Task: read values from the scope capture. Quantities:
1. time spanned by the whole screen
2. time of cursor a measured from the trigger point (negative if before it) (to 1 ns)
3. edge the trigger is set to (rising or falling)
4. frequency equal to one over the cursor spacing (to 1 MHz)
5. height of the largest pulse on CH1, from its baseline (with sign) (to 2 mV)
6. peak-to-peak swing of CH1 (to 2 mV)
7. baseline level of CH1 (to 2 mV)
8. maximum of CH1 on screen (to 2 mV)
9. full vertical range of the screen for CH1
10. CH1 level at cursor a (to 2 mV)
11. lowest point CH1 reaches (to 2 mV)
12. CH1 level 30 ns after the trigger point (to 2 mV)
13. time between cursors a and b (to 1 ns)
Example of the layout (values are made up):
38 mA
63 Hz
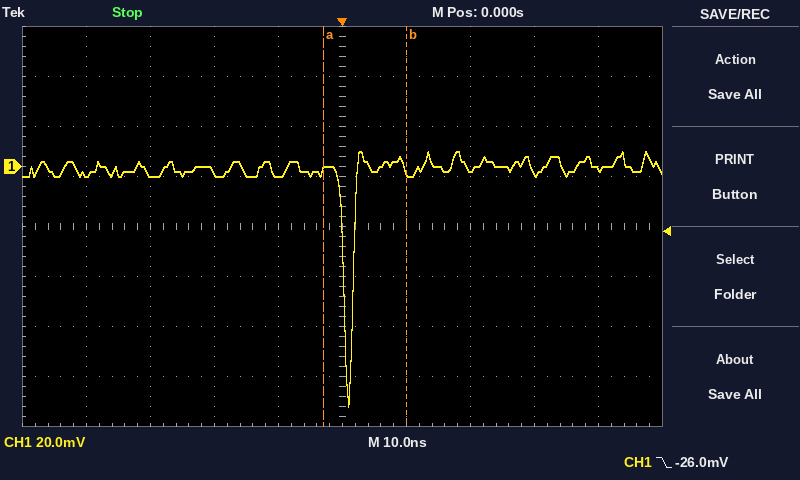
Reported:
100 ns
-3 ns
falling
77 MHz
-96 mV
102 mV
0 mV
6 mV
160 mV
-2 mV
-96 mV
-2 mV
13 ns
